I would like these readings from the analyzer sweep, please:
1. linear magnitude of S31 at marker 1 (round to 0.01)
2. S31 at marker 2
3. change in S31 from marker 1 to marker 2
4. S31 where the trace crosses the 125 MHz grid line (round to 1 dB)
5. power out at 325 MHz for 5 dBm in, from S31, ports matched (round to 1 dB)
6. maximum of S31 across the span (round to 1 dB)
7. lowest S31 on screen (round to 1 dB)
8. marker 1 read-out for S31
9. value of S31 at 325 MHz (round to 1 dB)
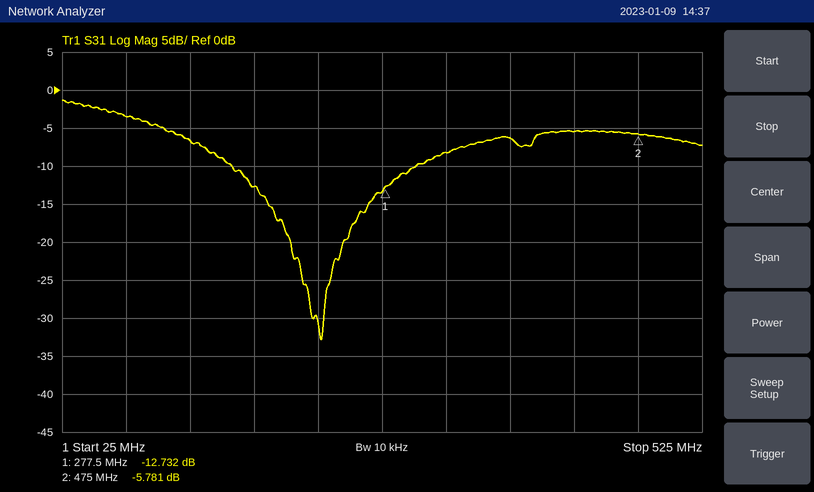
0.23
-5.781 dB
6.951 dB
-7 dB
-3 dBm
-1 dB
-33 dB
-12.732 dB
-8 dB
